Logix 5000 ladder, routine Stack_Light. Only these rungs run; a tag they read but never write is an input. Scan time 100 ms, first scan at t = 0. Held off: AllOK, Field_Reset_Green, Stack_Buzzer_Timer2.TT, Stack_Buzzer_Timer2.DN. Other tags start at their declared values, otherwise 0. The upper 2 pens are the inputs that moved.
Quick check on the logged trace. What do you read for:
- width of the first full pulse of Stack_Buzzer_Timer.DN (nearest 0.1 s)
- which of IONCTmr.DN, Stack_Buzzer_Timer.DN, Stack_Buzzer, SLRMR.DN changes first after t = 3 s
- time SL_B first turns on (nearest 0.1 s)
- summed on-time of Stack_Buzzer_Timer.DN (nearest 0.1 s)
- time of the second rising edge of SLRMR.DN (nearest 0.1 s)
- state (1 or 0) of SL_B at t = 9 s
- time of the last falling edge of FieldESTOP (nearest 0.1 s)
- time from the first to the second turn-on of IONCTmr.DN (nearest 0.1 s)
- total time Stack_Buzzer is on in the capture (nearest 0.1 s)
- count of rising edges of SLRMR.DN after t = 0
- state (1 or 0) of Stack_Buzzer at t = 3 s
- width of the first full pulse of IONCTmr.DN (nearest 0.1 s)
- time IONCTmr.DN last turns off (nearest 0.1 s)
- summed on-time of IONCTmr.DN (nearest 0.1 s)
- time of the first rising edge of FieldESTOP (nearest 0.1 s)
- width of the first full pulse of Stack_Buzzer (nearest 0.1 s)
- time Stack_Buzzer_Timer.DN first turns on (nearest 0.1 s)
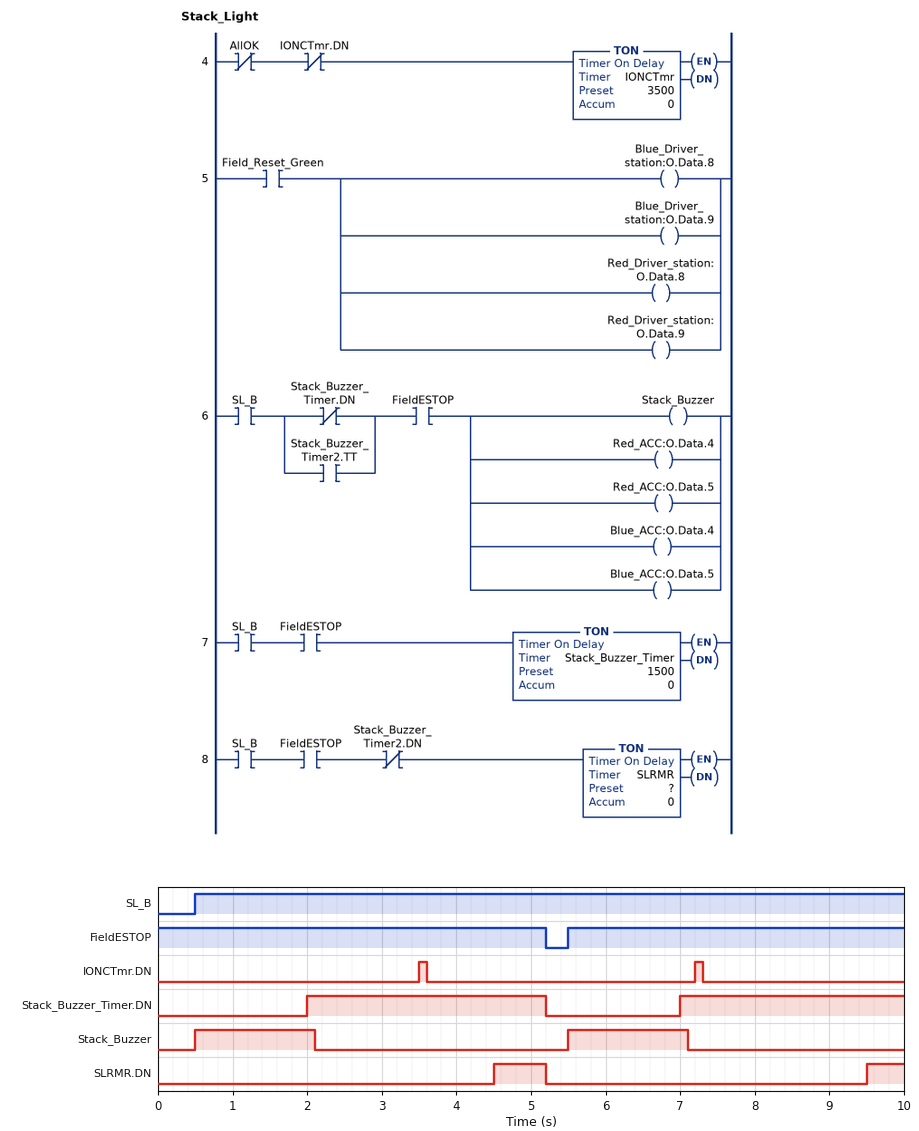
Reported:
3.2 s
IONCTmr.DN
0.5 s
6.2 s
9.5 s
1
5.2 s
3.7 s
3.2 s
2
0
0.1 s
7.3 s
0.2 s
5.5 s
1.6 s
2.0 s
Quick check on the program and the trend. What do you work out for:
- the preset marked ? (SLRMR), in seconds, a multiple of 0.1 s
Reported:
4.0 s
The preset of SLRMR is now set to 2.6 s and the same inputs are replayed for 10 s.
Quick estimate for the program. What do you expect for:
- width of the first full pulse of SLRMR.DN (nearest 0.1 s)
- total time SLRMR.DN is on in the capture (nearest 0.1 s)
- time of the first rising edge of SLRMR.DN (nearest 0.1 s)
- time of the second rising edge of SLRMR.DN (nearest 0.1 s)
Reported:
2.1 s
4.0 s
3.1 s
8.1 s
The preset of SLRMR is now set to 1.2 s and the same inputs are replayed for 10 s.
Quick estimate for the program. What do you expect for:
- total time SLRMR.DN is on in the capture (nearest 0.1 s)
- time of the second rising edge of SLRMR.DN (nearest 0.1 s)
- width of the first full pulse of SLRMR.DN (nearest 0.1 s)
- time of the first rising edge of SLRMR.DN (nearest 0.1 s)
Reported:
6.8 s
6.7 s
3.5 s
1.7 s
